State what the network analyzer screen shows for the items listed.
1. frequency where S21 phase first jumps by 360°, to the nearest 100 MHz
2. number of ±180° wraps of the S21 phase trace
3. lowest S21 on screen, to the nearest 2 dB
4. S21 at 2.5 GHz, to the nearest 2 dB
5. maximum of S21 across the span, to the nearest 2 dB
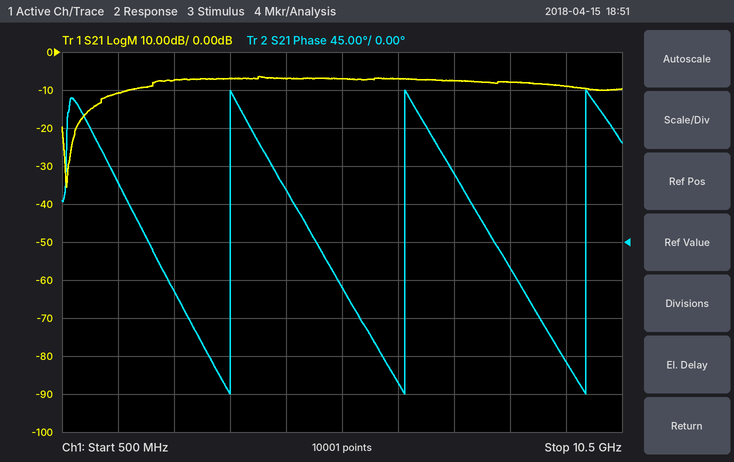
3.5 GHz
3
-36 dB
-8 dB
-6 dB
